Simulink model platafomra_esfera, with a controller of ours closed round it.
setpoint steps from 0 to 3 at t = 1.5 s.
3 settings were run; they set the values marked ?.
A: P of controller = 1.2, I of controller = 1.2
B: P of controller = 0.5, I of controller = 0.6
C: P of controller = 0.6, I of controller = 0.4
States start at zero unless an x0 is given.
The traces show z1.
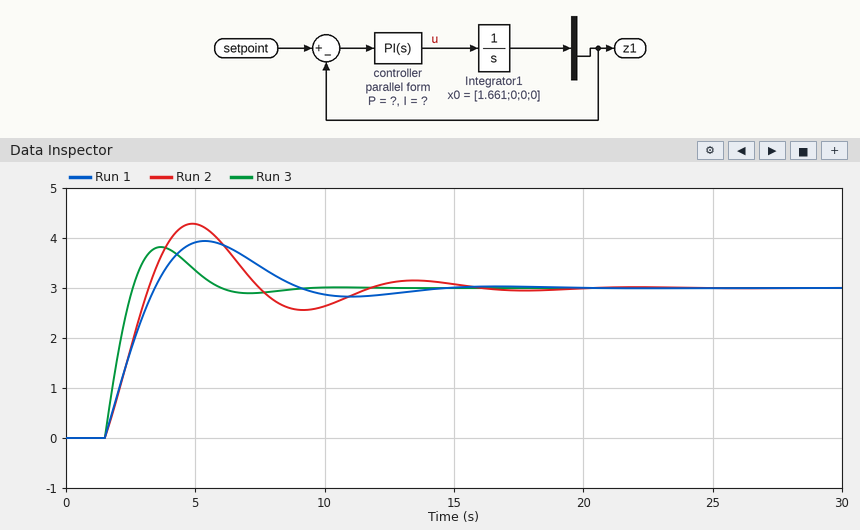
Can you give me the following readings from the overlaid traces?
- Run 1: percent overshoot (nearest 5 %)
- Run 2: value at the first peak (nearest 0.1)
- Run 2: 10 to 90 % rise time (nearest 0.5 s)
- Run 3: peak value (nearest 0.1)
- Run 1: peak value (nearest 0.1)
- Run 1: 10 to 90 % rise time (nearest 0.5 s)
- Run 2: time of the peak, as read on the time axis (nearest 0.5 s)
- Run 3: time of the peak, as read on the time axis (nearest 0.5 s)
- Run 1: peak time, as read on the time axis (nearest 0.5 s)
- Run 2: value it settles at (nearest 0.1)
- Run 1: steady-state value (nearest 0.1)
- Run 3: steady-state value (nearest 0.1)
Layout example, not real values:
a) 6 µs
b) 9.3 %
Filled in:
a) 30 %
b) 4.3
c) 1.5 s
d) 3.8
e) 3.9
f) 1.5 s
g) 5.0 s
h) 3.5 s
i) 5.5 s
j) 3.0
k) 3.0
l) 3.0
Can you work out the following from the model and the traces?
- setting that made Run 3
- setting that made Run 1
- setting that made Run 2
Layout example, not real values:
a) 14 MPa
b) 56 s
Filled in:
a) A
b) C
c) B
